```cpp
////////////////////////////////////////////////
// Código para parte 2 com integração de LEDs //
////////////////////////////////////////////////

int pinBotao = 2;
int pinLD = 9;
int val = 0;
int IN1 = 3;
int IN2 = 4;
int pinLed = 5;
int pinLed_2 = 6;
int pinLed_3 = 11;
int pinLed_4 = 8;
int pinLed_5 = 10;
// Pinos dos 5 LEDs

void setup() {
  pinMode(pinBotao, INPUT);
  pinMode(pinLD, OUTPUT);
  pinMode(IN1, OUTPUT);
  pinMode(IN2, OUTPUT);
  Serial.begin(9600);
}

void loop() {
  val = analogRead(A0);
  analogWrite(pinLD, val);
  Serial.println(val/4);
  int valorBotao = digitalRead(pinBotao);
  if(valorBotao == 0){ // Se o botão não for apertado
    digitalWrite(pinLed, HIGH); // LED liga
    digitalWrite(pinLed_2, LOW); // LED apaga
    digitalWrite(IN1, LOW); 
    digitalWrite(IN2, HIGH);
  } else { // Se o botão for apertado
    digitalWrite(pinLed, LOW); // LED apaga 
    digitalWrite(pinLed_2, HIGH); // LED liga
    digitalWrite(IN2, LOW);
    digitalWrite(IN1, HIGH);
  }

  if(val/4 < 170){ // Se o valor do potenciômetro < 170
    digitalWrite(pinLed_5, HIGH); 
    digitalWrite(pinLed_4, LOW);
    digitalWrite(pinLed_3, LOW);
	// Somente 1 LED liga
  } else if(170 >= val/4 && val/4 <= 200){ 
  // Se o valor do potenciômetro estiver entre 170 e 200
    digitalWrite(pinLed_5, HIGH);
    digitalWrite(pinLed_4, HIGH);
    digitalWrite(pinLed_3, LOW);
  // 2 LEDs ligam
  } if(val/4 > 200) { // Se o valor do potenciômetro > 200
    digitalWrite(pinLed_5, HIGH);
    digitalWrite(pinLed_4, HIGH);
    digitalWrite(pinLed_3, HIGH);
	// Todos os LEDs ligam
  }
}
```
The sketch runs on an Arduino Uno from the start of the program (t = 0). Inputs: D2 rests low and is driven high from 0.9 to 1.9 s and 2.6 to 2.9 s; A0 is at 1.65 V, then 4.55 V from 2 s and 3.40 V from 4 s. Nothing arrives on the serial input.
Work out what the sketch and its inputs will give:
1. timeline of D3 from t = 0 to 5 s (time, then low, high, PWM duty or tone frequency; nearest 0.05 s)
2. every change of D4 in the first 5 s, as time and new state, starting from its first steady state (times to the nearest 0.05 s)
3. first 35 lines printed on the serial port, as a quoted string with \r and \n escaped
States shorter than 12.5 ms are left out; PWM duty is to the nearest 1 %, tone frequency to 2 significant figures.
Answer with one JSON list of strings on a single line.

["0 s low; 0.9 s high; 1.9 s low; 2.6 s high; 2.9 s low", "0 s high; 0.9 s low; 1.9 s high; 2.6 s low; 2.9 s high", "\"84\\r\\n84\\r\\n84\\r\\n84\\r\\n84\\r\\n84\\r\\n84\\r\\n84\\r\\n84\\r\\n84\\r\\n84\\r\\n84\\r\\n84\\r\\n84\\r\\n84\\r\\n84\\r\\n84\\r\\n84\\r\\n84\\r\\n84\\r\\n84\\r\\n84\\r\\n84\\r\\n84\\r\\n84\\r\\n84\\r\\n84\\r\\n84\\r\\n84\\r\\n84\\r\\n84\\r\\n84\\r\\n84\\r\\n84\\r\\n84\\r\\n\""]
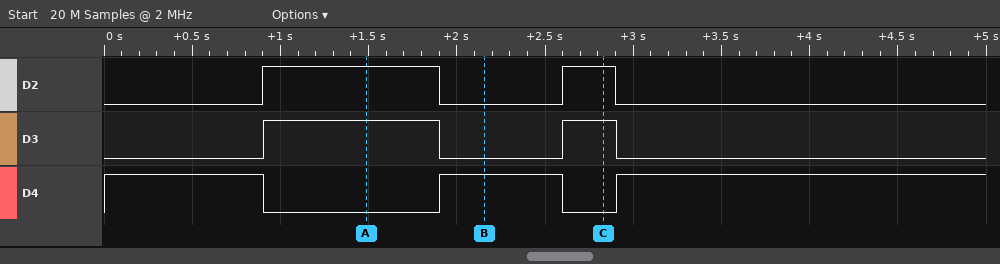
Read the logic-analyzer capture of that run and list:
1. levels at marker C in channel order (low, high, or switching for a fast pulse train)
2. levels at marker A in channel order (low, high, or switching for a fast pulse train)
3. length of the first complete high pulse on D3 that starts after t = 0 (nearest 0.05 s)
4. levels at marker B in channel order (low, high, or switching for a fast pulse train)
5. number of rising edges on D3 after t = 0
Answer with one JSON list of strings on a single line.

["D2 high, D3 high, D4 low", "D2 high, D3 high, D4 low", "1.00 s", "D2 low, D3 low, D4 high", "2"]
